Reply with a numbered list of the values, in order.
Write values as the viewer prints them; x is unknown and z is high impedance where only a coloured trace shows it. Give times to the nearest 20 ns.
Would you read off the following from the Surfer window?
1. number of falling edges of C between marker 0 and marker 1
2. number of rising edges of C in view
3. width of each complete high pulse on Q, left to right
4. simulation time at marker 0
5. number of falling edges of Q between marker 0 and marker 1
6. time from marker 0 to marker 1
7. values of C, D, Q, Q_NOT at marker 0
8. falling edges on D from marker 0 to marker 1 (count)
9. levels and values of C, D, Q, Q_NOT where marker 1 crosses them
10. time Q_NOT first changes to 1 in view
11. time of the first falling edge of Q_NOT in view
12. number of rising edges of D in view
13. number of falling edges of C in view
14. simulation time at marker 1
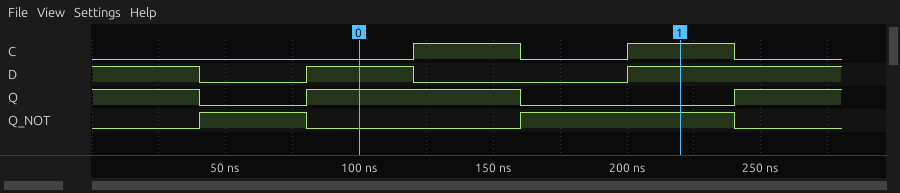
1. 1
2. 2
3. 80 ns
4. 100 ns
5. 1
6. 120 ns
7. C=0, D=1, Q=1, Q_NOT=0
8. 1
9. C=1, D=1, Q=0, Q_NOT=1
10. 40 ns
11. 80 ns
12. 2
13. 2
14. 220 ns
